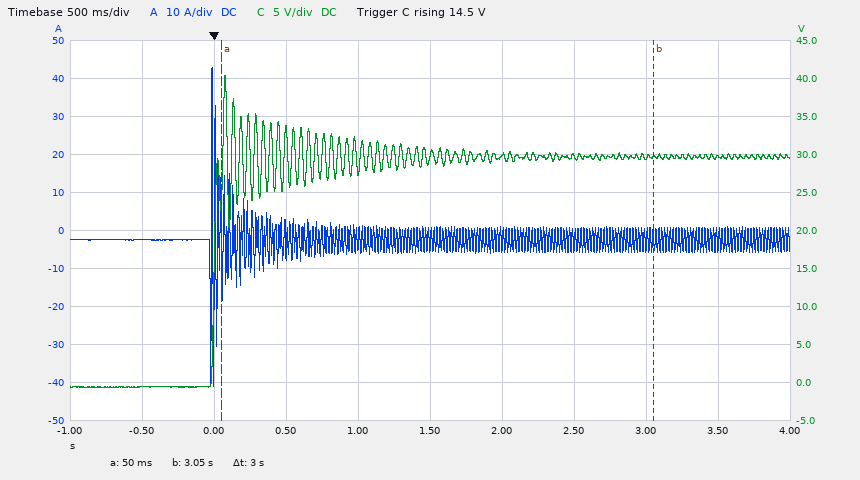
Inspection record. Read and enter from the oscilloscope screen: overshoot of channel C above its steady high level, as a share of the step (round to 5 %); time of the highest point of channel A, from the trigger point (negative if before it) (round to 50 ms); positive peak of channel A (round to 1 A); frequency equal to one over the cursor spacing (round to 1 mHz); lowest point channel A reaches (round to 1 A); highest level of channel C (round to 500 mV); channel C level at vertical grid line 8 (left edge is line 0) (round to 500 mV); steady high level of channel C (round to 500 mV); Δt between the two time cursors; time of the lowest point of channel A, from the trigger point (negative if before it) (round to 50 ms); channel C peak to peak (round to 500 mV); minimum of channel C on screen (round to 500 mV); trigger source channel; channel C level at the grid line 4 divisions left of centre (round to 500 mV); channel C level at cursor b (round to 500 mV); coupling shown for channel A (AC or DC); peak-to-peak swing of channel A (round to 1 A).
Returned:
35 %
0 ms
43 A
333 mHz
-41 A
40.5 V
29.5 V
29.5 V
3 s
0 ms
41.0 V
-500 mV
channel C
-500 mV
29.5 V
DC
84 A
